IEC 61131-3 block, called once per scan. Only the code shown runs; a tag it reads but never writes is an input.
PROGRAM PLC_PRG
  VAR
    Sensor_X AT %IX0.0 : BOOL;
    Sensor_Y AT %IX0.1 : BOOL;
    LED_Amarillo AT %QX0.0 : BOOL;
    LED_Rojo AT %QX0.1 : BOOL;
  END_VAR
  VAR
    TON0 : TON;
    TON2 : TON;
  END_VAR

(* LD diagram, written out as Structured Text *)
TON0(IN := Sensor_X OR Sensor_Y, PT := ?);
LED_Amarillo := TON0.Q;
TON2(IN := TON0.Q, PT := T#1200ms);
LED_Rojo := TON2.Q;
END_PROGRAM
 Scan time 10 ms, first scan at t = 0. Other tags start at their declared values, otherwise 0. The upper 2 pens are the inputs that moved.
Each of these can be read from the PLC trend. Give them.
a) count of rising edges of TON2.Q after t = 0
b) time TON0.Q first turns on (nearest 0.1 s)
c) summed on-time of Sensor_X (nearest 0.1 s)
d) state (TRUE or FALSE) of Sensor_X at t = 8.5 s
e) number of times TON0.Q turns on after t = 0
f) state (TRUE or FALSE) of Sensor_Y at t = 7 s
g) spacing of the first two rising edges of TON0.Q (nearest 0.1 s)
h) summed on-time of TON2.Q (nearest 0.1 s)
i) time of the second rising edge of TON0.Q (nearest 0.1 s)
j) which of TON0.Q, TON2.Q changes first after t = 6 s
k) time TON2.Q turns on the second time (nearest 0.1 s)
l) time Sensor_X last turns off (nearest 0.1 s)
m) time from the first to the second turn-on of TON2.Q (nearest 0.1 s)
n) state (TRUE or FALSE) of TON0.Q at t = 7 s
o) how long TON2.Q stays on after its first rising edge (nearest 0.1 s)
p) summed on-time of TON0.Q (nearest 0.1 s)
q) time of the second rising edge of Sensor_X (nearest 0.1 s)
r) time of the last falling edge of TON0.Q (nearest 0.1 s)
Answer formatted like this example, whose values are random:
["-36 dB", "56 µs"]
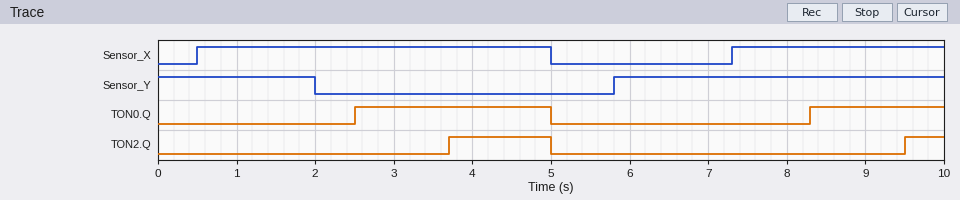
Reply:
["2", "2.5 s", "7.2 s", "TRUE", "2", "TRUE", "5.8 s", "1.8 s", "8.3 s", "TON0.Q", "9.5 s", "5.0 s", "5.8 s", "FALSE", "1.3 s", "4.2 s", "7.3 s", "5.0 s"]
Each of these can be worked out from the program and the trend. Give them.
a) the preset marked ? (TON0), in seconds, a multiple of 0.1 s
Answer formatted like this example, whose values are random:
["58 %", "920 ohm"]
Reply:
["2.5 s"]
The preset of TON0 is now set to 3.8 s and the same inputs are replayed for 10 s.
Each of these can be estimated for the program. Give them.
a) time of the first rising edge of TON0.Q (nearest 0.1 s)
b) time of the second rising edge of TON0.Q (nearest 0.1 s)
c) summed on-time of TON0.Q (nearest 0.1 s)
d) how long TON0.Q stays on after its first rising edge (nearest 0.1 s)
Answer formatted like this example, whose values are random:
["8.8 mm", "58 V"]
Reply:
["3.8 s", "9.6 s", "1.6 s", "1.2 s"]
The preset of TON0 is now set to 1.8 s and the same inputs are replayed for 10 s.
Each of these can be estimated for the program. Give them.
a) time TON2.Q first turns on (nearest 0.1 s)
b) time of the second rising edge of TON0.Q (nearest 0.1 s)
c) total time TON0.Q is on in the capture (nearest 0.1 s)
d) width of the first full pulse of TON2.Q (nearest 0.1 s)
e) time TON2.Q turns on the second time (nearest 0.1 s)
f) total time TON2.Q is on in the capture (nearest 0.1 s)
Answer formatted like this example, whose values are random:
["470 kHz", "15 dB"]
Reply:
["3.0 s", "7.6 s", "5.6 s", "2.0 s", "8.8 s", "3.2 s"]
